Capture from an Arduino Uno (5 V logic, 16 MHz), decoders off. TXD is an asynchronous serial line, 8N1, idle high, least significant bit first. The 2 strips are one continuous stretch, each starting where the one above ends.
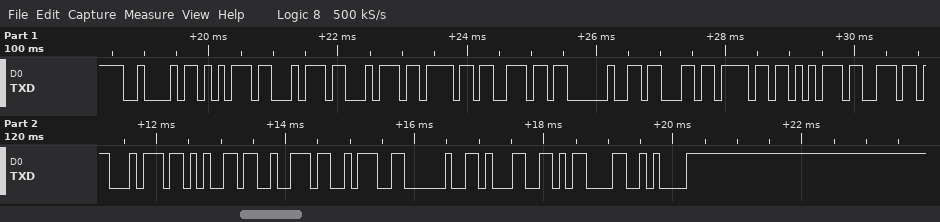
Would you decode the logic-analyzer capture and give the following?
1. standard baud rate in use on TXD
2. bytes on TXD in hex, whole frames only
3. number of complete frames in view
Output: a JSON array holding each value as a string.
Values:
["9600 baud", "0x42 0x75 0x74 0x74 0x6F 0x6E 0x20 0x63 0x6F 0x75 0x6E 0x74 0x65 0x72 0x3A 0x20 0x31 0x0D 0x0A", "19"]
